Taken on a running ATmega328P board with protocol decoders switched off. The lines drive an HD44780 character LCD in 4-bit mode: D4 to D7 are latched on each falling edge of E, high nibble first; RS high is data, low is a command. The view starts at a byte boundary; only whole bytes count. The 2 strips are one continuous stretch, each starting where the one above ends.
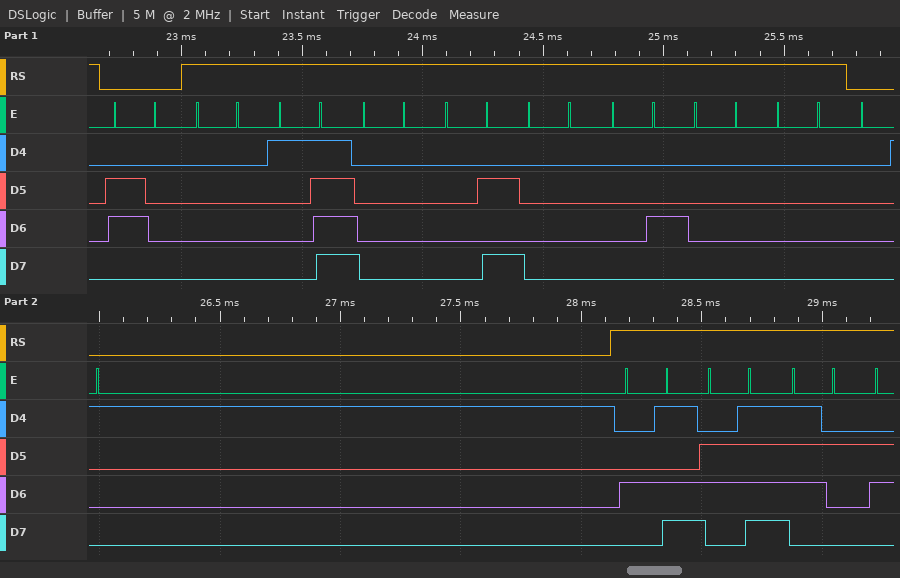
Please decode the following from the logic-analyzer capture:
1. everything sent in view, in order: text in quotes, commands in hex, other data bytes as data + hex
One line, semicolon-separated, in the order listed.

0x60 data 00 1F 00 0A 00 04 00 00 0x01 "Mor"
